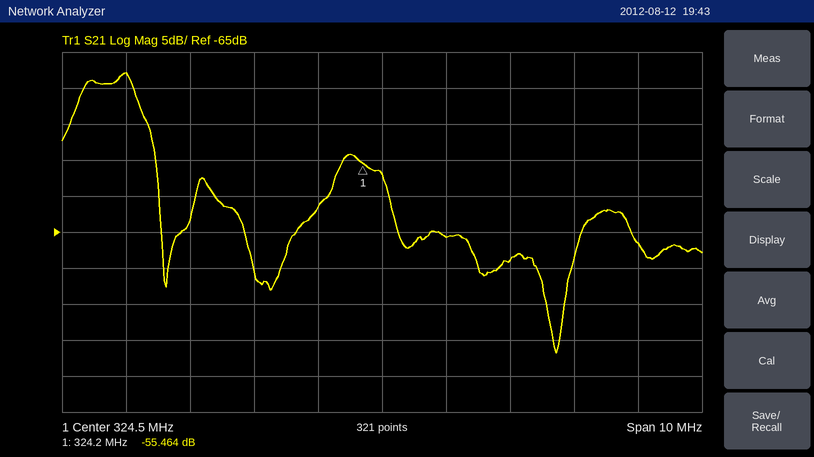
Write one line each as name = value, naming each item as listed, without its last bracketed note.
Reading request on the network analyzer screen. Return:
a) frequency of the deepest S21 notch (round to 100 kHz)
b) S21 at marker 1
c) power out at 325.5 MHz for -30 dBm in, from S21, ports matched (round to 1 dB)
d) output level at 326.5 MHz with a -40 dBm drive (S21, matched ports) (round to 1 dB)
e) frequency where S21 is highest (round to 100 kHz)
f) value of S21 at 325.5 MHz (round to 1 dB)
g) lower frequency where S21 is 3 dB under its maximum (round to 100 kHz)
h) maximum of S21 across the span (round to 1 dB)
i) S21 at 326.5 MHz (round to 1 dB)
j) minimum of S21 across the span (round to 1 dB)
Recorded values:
frequency of the deepest S21 notch = 327.2 MHz
S21 at marker 1 = -55.464 dB
power out at 325.5 MHz for -30 dBm in, from S21, ports matched = -96 dBm
output level at 326.5 MHz with a -40 dBm drive (S21, matched ports) = -109 dBm
frequency where S21 is highest = 320.5 MHz
value of S21 at 325.5 MHz = -66 dB
lower frequency where S21 is 3 dB under its maximum = 319.8 MHz
maximum of S21 across the span = -43 dB
S21 at 326.5 MHz = -69 dB
minimum of S21 across the span = -82 dB
